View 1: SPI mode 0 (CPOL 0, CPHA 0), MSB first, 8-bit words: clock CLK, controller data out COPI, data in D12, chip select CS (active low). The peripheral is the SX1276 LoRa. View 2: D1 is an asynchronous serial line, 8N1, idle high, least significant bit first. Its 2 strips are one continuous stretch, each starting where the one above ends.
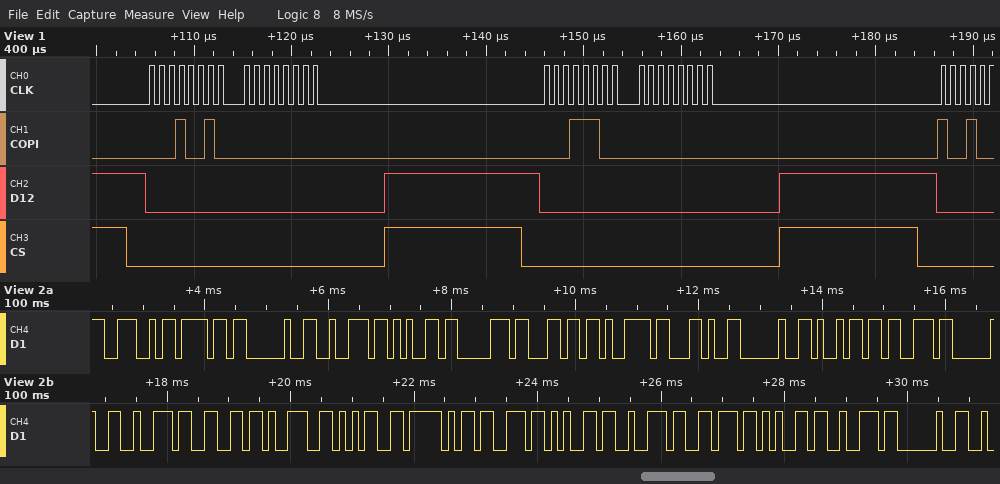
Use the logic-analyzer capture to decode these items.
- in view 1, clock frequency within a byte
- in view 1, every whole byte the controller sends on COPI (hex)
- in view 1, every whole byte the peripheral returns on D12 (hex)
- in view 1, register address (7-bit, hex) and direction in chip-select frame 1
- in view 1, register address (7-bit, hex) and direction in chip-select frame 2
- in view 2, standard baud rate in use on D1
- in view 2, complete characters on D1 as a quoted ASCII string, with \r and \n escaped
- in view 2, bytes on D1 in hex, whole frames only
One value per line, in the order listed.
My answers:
1 MHz
12 00 1C 00
00 00 00 00
0x12 read
0x1C read
9600 baud
"No reply, is rf95_server "
4E 6F 20 72 65 70 6C 79 2C 20 69 73 20 72 66 39 35 5F 73 65 72 76 65 72 20
